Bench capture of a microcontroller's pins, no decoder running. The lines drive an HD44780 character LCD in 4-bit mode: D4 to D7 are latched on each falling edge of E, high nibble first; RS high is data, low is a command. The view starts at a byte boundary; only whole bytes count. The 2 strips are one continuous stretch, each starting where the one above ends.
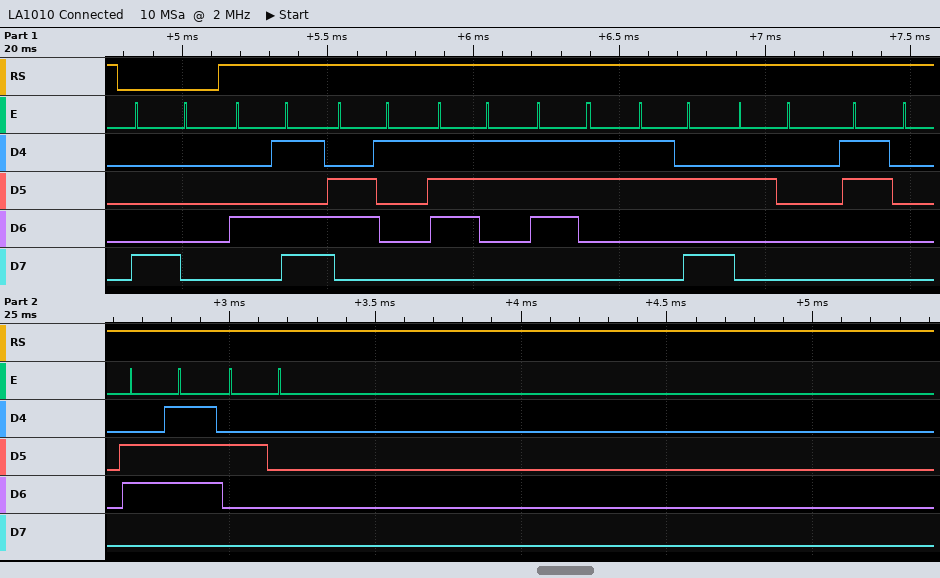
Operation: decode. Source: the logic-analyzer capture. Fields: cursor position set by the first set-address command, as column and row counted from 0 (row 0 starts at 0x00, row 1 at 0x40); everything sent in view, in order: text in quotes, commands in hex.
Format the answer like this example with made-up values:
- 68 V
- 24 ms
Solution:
- column 0, row 0
- 0x80 "Mass: 0g "
